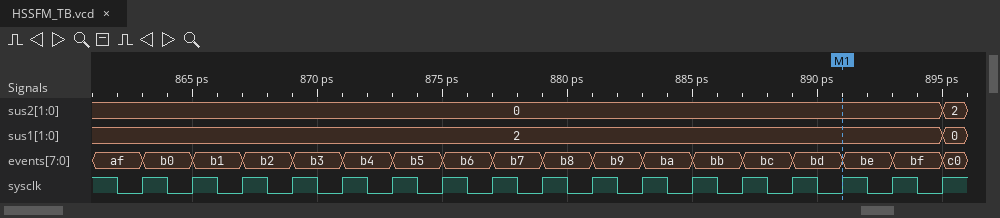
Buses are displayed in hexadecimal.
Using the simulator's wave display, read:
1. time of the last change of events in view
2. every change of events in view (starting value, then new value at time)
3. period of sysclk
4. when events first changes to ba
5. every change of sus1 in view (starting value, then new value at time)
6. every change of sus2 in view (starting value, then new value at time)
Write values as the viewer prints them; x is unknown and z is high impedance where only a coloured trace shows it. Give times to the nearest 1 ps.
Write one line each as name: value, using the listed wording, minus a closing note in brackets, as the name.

time of the last change of events in view: 895 ps
every change of events in view: af, b0 at 863 ps, b1 at 865 ps, b2 at 867 ps, b3 at 869 ps, b4 at 871 ps, b5 at 873 ps, b6 at 875 ps, b7 at 877 ps, b8 at 879 ps, b9 at 881 ps, ba at 883 ps, bb at 885 ps, bc at 887 ps, bd at 889 ps, be at 891 ps, bf at 893 ps, c0 at 895 ps
period of sysclk: 2 ps
when events first changes to ba: 883 ps
every change of sus1 in view: 2, 0 at 895 ps
every change of sus2 in view: 0, 2 at 895 ps
